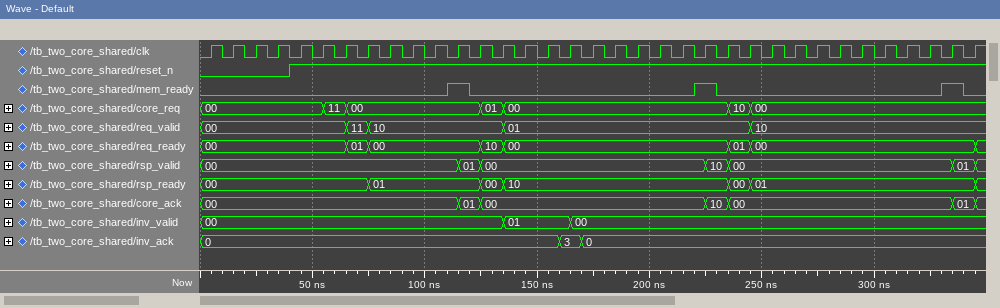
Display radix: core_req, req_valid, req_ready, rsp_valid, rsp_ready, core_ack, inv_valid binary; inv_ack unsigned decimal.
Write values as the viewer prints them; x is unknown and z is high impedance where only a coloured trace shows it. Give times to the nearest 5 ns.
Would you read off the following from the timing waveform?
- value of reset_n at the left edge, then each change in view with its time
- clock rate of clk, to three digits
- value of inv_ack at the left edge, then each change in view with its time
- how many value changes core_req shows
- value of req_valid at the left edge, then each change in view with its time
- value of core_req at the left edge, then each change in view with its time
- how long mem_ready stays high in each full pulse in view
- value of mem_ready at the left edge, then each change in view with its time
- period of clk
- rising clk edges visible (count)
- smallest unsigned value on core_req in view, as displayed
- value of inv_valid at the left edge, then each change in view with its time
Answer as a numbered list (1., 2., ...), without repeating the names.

1. 0, 1 at 40 ns
2. 100 MHz
3. 0, 3 at 160 ns, 0 at 170 ns
4. 6
5. 00, 11 at 65 ns, 10 at 75 ns, 01 at 135 ns, 10 at 245 ns
6. 00, 11 at 55 ns, 00 at 65 ns, 01 at 125 ns, 00 at 135 ns, 10 at 235 ns, 00 at 245 ns
7. 10 ns, 10 ns, 10 ns
8. 0, 1 at 110 ns, 0 at 120 ns, 1 at 220 ns, 0 at 230 ns, 1 at 330 ns, 0 at 340 ns
9. 10 ns
10. 35
11. 00
12. 00, 01 at 135 ns, 00 at 165 ns
